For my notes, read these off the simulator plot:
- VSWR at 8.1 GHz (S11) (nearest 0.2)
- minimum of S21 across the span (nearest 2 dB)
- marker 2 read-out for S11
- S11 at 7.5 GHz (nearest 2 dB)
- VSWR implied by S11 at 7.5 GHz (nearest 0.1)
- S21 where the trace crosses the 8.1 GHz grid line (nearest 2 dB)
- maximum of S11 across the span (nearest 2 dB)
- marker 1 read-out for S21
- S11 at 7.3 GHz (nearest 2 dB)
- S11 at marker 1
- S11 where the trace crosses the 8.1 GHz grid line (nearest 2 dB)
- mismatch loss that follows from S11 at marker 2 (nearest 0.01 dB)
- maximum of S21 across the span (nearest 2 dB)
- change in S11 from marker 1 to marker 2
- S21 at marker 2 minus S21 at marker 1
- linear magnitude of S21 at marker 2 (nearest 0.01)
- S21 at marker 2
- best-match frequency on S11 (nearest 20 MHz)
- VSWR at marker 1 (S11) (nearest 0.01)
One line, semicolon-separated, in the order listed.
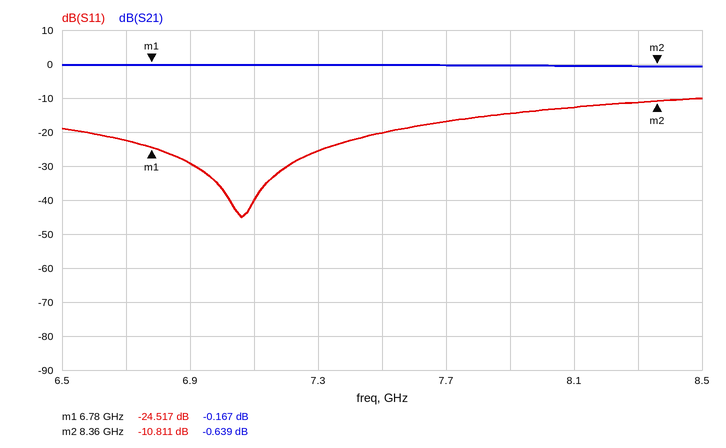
1.6; 0 dB; -10.811 dB; -20 dB; 1.2; 0 dB; -10 dB; -0.167 dB; -26 dB; -24.517 dB; -12 dB; 0.38 dB; 0 dB; 13.706 dB; -0.472 dB; 0.93; -0.639 dB; 7.06 GHz; 1.13
